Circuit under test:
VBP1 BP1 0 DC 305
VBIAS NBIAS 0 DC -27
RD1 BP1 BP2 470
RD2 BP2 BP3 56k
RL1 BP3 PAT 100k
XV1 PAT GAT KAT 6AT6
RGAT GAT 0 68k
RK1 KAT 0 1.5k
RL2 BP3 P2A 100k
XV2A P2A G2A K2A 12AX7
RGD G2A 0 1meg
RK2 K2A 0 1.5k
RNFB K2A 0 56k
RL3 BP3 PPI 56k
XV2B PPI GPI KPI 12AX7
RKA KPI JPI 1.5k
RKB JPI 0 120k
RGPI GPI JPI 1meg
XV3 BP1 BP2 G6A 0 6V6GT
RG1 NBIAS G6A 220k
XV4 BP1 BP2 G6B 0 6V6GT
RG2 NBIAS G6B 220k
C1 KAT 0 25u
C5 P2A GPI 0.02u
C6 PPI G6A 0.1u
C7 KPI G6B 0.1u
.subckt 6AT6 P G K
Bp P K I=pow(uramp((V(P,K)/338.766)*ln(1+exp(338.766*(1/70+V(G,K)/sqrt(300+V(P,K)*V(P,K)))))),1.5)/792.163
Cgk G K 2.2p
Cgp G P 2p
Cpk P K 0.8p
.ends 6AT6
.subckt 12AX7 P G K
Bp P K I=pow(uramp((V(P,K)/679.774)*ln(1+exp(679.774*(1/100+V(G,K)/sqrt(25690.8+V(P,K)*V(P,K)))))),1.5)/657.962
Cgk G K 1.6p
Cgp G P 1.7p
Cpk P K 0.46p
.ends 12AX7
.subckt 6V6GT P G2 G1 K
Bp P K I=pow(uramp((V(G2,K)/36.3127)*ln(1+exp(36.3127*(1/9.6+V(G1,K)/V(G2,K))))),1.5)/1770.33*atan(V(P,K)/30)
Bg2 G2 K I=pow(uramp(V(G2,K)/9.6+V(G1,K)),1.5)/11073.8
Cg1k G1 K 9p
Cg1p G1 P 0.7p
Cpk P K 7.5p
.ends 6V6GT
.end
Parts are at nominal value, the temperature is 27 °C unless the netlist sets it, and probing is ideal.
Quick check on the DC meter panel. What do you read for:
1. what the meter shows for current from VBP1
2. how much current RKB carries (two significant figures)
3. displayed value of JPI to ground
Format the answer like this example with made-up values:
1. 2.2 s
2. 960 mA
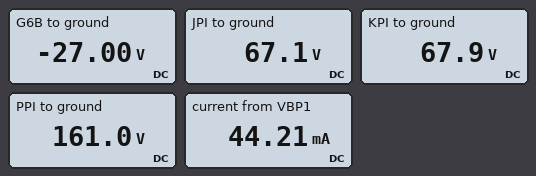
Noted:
1. 44.21 mA
2. 560 µA
3. 67.1 V
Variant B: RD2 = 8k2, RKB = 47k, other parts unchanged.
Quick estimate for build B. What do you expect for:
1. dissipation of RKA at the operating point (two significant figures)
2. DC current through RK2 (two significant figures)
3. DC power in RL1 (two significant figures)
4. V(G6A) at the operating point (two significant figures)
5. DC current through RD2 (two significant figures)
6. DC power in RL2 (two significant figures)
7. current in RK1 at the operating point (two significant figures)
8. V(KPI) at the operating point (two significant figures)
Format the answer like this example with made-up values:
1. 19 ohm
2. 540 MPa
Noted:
1. 1.4 mW
2. 950 µA
3. 120 mW
4. -27 V
5. 3.0 mA
6. 95 mW
7. 1.1 mA
8. 46 V
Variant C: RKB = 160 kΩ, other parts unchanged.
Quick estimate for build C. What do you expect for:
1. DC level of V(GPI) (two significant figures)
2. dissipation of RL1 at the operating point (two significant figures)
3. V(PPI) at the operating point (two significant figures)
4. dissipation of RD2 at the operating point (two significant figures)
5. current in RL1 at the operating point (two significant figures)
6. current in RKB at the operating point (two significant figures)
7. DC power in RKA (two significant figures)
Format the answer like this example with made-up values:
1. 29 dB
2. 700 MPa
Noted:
1. 82 V
2. 53 mW
3. 170 V
4. 210 mW
5. 730 µA
6. 510 µA
7. 390 µW
